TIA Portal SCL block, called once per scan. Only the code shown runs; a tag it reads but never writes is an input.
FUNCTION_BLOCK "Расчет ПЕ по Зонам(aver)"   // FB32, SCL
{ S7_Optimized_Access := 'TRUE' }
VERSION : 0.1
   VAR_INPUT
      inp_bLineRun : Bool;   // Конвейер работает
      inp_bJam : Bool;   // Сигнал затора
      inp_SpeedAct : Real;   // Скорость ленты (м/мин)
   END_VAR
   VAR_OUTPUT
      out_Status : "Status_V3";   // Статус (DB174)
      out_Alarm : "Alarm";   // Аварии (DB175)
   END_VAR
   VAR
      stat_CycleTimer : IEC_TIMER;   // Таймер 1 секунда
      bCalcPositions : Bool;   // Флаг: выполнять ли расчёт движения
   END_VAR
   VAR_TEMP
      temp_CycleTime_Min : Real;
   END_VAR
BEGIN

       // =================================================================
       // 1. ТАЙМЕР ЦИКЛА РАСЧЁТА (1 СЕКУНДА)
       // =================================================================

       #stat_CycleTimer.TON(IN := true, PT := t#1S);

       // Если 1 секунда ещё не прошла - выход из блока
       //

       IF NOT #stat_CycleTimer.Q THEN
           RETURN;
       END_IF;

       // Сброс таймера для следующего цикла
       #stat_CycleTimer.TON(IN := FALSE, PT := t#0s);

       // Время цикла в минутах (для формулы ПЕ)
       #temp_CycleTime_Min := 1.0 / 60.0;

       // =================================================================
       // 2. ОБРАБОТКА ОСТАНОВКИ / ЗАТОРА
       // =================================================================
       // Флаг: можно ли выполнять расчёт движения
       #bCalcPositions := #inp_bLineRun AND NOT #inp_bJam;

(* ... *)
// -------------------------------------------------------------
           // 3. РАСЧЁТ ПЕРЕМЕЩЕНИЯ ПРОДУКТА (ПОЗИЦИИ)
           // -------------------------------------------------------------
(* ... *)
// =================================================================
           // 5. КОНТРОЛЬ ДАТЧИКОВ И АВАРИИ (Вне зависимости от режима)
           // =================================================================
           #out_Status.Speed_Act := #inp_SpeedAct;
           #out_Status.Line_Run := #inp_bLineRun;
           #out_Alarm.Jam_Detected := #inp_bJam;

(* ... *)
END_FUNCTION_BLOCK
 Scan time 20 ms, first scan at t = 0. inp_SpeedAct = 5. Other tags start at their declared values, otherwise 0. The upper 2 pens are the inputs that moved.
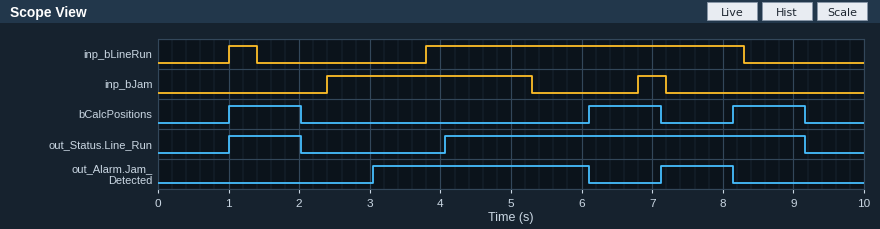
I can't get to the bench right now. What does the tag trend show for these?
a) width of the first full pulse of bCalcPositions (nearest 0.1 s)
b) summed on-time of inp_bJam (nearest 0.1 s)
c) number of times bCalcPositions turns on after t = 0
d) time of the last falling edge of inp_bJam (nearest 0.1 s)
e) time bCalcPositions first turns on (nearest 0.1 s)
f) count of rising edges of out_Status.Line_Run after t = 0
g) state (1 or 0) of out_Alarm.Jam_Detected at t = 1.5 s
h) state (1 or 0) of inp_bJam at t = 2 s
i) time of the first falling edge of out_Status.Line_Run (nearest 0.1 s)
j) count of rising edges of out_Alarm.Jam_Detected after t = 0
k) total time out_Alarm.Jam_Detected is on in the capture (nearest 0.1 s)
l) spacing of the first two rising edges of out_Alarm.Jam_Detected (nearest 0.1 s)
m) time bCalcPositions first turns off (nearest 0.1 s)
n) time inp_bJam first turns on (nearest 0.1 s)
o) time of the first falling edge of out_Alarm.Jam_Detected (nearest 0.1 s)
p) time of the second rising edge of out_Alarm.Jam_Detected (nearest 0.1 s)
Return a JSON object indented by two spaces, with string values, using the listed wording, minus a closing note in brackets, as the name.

{
  "width of the first full pulse of bCalcPositions": "1.0 s",
  "summed on-time of inp_bJam": "3.3 s",
  "number of times bCalcPositions turns on after t = 0": "3",
  "time of the last falling edge of inp_bJam": "7.2 s",
  "time bCalcPositions first turns on": "1.0 s",
  "count of rising edges of out_Status.Line_Run after t = 0": "2",
  "state (1 or 0) of out_Alarm.Jam_Detected at t = 1.5 s": "0",
  "state (1 or 0) of inp_bJam at t = 2 s": "0",
  "time of the first falling edge of out_Status.Line_Run": "2.0 s",
  "count of rising edges of out_Alarm.Jam_Detected after t = 0": "2",
  "total time out_Alarm.Jam_Detected is on in the capture": "4.1 s",
  "spacing of the first two rising edges of out_Alarm.Jam_Detected": "4.1 s",
  "time bCalcPositions first turns off": "2.0 s",
  "time inp_bJam first turns on": "2.4 s",
  "time of the first falling edge of out_Alarm.Jam_Detected": "6.1 s",
  "time of the second rising edge of out_Alarm.Jam_Detected": "7.1 s"
}
